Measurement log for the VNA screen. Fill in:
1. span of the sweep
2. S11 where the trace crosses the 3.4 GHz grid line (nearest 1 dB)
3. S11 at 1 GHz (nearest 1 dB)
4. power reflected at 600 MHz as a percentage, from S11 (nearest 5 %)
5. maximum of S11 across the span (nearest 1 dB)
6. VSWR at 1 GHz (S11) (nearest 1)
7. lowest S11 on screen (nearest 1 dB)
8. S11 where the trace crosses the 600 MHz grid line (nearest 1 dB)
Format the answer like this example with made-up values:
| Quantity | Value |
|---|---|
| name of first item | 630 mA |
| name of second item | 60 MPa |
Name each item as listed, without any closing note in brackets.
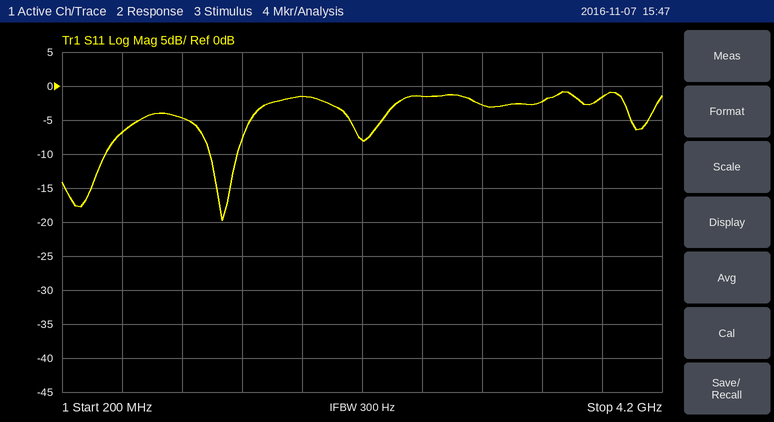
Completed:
| Quantity | Value |
|---|---|
| span of the sweep | 4 GHz |
| S11 where the trace crosses the 3.4 GHz grid line | -2 dB |
| S11 at 1 GHz | -5 dB |
| power reflected at 600 MHz as a percentage, from S11 | 20 % |
| maximum of S11 across the span | -1 dB |
| VSWR at 1 GHz (S11) | 4 |
| lowest S11 on screen | -20 dB |
| S11 where the trace crosses the 600 MHz grid line | -7 dB |
